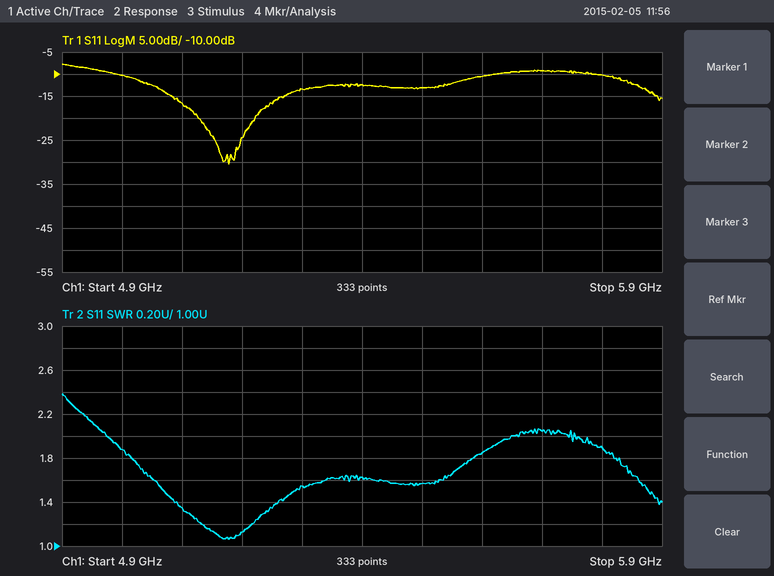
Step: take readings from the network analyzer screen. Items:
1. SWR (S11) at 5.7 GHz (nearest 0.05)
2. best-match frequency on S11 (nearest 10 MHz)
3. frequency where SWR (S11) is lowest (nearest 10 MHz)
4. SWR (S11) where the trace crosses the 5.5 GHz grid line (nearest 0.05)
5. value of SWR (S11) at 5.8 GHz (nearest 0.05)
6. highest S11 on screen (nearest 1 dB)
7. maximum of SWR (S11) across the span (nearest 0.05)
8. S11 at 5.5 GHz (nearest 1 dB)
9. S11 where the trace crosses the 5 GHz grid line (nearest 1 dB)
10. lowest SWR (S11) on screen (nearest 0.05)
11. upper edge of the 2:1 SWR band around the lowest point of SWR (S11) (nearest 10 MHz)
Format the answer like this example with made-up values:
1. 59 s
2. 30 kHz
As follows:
1. 2.05
2. 5.18 GHz
3. 5.18 GHz
4. 1.55
5. 1.90
6. -8 dB
7. 2.40
8. -13 dB
9. -10 dB
10. 1.05
11. 5.65 GHz
